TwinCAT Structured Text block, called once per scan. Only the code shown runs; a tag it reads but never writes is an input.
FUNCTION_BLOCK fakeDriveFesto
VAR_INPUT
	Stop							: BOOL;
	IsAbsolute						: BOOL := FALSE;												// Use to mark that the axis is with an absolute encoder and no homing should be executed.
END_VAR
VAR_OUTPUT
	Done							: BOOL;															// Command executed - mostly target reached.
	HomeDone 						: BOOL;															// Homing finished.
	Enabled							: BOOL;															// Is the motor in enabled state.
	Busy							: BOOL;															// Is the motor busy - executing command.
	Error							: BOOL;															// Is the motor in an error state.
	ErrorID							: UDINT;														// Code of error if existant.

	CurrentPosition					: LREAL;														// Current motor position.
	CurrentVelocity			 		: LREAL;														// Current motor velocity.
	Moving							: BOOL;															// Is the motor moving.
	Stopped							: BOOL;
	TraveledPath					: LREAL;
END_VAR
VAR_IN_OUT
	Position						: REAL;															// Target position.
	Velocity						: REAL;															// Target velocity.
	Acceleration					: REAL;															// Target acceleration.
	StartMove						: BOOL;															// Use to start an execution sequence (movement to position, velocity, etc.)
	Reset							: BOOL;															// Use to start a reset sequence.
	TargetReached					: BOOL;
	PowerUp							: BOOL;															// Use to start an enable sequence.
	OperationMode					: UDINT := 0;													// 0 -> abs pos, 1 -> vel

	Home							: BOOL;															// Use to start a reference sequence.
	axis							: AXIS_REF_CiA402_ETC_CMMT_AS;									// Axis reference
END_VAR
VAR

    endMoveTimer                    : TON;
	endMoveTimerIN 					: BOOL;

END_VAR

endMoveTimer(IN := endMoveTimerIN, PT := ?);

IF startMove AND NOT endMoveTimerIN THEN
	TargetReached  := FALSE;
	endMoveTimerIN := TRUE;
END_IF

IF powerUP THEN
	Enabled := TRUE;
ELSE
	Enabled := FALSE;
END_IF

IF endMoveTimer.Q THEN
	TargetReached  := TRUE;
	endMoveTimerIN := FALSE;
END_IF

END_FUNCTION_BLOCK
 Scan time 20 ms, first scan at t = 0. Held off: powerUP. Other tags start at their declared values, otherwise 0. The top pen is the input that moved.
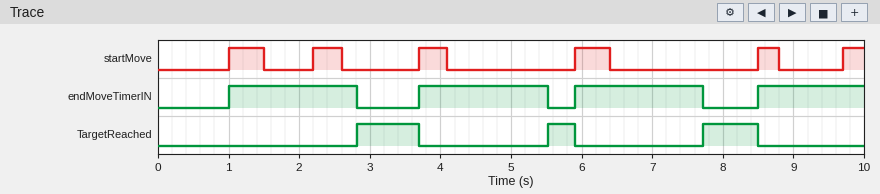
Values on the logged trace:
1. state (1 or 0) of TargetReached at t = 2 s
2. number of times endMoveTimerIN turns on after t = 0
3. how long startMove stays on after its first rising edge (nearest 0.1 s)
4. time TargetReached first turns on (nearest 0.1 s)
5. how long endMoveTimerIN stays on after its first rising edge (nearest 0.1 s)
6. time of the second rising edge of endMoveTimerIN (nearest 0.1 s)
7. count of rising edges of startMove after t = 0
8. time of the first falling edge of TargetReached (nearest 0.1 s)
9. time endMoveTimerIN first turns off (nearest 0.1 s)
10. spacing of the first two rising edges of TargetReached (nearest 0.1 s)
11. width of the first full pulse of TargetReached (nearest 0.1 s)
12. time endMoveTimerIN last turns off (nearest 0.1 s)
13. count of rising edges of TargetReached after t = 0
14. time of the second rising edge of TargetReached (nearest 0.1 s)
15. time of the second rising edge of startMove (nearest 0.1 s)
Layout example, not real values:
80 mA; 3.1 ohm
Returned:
0; 4; 0.5 s; 2.8 s; 1.8 s; 3.7 s; 6; 3.7 s; 2.8 s; 2.7 s; 0.9 s; 7.7 s; 3; 5.5 s; 2.2 s
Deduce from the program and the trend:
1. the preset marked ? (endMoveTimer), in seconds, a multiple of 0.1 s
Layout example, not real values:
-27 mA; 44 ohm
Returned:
1.8 s
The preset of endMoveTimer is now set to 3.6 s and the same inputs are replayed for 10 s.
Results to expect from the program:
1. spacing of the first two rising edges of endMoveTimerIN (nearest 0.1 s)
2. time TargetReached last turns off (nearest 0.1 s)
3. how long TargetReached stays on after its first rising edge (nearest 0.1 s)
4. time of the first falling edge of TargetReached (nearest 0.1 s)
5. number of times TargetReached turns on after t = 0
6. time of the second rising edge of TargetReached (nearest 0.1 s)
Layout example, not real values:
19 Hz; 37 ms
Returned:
4.9 s; 9.7 s; 1.3 s; 5.9 s; 2; 9.5 s
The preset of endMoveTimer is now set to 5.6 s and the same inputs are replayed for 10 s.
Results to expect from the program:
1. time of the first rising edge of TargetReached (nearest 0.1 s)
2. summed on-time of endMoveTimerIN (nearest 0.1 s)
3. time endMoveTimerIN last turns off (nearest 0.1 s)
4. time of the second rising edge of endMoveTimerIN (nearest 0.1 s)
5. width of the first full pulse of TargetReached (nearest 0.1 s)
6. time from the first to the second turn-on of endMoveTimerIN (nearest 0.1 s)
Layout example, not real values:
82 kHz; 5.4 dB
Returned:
6.6 s; 7.1 s; 6.6 s; 8.5 s; 1.9 s; 7.5 s
